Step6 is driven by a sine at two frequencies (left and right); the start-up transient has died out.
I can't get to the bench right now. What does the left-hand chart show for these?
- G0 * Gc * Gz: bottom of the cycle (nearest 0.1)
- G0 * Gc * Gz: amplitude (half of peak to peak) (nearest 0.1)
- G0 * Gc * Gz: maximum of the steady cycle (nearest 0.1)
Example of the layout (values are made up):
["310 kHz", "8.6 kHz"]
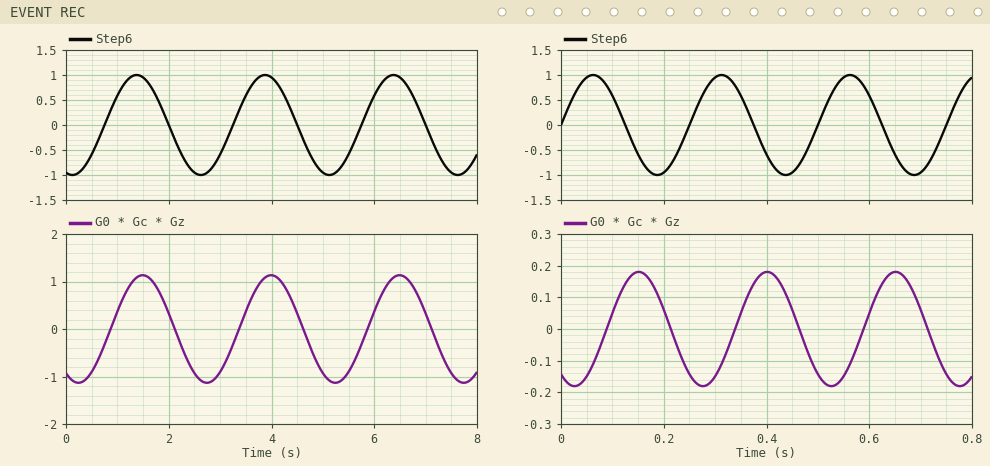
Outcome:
["-1.1", "1.1", "1.1"]
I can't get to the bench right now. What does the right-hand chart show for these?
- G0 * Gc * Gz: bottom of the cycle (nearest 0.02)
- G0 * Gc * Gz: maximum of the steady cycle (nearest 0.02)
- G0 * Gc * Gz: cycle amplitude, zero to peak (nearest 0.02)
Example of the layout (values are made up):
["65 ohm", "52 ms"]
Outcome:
["-0.18", "0.18", "0.18"]
